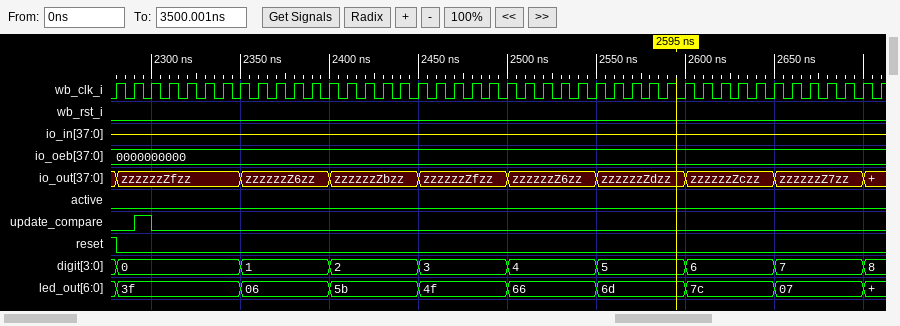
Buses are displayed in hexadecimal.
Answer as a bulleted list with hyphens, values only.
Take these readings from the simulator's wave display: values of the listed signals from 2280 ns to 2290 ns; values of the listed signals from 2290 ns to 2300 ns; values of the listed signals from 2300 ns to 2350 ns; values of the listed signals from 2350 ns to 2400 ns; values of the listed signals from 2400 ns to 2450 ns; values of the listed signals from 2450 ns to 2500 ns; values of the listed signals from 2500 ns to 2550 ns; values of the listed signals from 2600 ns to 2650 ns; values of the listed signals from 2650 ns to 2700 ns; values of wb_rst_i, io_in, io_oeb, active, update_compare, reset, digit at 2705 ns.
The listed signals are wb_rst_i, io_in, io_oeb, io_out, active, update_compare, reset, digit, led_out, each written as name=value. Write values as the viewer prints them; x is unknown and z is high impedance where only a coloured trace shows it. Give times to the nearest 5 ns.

- wb_rst_i=0, io_in=z, io_oeb=0000000000, io_out=zzzzzzZfzz, active=0, update_compare=0, reset=0, digit=0, led_out=3f
- wb_rst_i=0, io_in=z, io_oeb=0000000000, io_out=zzzzzzZfzz, active=0, update_compare=1, reset=0, digit=0, led_out=3f
- wb_rst_i=0, io_in=z, io_oeb=0000000000, io_out=zzzzzzZfzz, active=0, update_compare=0, reset=0, digit=0, led_out=3f
- wb_rst_i=0, io_in=z, io_oeb=0000000000, io_out=zzzzzzZ6zz, active=0, update_compare=0, reset=0, digit=1, led_out=06
- wb_rst_i=0, io_in=z, io_oeb=0000000000, io_out=zzzzzzZbzz, active=0, update_compare=0, reset=0, digit=2, led_out=5b
- wb_rst_i=0, io_in=z, io_oeb=0000000000, io_out=zzzzzzZfzz, active=0, update_compare=0, reset=0, digit=3, led_out=4f
- wb_rst_i=0, io_in=z, io_oeb=0000000000, io_out=zzzzzzZ6zz, active=0, update_compare=0, reset=0, digit=4, led_out=66
- wb_rst_i=0, io_in=z, io_oeb=0000000000, io_out=zzzzzzZczz, active=0, update_compare=0, reset=0, digit=6, led_out=7c
- wb_rst_i=0, io_in=z, io_oeb=0000000000, io_out=zzzzzzZ7zz, active=0, update_compare=0, reset=0, digit=7, led_out=07
- wb_rst_i=0, io_in=z, io_oeb=0000000000, active=0, update_compare=0, reset=0, digit=8
